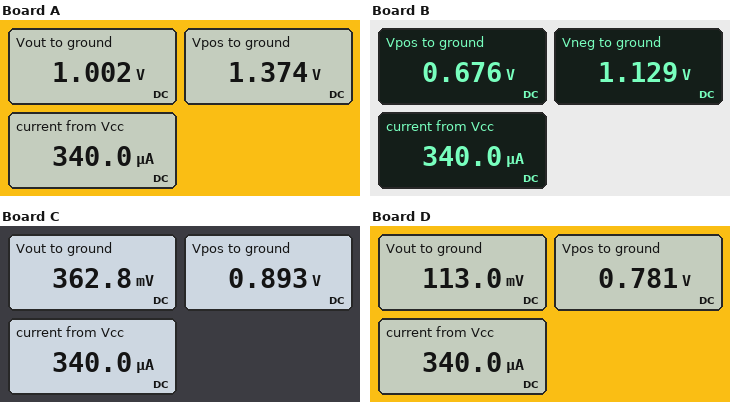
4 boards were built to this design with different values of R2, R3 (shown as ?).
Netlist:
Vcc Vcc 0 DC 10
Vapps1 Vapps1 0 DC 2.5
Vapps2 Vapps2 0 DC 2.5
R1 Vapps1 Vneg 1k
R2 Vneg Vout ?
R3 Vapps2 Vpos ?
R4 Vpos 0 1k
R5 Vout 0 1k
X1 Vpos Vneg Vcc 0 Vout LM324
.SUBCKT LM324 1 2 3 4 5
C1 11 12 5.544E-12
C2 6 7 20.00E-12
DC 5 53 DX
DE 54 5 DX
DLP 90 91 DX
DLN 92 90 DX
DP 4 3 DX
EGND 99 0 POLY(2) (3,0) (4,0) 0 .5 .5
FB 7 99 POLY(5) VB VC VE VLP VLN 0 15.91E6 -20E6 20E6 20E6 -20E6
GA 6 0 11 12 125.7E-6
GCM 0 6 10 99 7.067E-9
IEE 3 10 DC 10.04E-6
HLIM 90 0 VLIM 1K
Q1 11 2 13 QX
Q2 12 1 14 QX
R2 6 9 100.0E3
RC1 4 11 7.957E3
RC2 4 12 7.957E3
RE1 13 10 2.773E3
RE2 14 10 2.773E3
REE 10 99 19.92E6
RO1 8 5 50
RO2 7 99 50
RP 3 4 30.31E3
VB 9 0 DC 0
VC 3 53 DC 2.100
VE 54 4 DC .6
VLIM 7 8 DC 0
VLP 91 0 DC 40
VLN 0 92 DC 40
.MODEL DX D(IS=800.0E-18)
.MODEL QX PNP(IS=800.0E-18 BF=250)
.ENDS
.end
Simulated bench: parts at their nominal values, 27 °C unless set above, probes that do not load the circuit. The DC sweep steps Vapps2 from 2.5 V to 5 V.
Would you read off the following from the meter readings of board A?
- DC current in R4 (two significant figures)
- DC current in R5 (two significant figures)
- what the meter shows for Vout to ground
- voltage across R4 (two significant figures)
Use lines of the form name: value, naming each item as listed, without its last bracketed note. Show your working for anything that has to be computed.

DC current in R4: (1.374 V) / 1 kΩ = 1.4 mA
DC current in R5: (1.002 V) / 1 kΩ = 1.0 mA
what the meter shows for Vout to ground: 1.002 V
voltage across R4: 1.374 V = 1.4 V
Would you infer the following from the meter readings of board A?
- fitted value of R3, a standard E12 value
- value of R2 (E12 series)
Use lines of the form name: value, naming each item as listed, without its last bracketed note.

fitted value of R3, a standard E12 value: 820 Ω
value of R2: 330 Ω
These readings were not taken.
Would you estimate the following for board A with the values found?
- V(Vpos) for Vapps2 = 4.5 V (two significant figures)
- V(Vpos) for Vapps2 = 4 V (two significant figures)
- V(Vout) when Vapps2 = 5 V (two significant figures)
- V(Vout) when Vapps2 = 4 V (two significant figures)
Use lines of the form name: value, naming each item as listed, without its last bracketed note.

V(Vpos) for Vapps2 = 4.5 V: 2.5 V
V(Vpos) for Vapps2 = 4 V: 2.2 V
V(Vout) when Vapps2 = 5 V: 2.8 V
V(Vout) when Vapps2 = 4 V: 2.1 V
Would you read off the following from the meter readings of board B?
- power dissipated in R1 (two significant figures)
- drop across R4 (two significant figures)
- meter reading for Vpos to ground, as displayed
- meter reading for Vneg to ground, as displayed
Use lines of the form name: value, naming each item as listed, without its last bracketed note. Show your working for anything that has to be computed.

power dissipated in R1: (2.5 V - 1.129 V)^2 / 1 kΩ = 1.9 mW
drop across R4: 676 mV = 680 mV
meter reading for Vpos to ground, as displayed: 0.676 V
meter reading for Vneg to ground, as displayed: 1.129 V
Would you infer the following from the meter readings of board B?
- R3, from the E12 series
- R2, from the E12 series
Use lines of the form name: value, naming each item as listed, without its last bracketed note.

R3, from the E12 series: 2.7 kΩ
R2, from the E12 series: 820 Ω
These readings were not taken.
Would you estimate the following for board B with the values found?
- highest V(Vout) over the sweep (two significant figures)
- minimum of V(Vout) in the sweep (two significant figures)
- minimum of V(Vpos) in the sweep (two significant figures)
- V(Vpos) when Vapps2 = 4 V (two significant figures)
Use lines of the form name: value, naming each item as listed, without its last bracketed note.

highest V(Vout) over the sweep: 410 mV
minimum of V(Vout) in the sweep: 4.2 mV
minimum of V(Vpos) in the sweep: 680 mV
V(Vpos) when Vapps2 = 4 V: 1.1 V
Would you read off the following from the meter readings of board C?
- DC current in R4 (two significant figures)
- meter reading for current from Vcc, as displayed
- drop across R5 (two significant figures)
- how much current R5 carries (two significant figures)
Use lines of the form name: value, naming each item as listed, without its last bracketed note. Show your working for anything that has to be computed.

DC current in R4: (893 mV) / 1 kΩ = 890 µA
meter reading for current from Vcc, as displayed: 340.0 µA
drop across R5: 362.8 mV = 360 mV
how much current R5 carries: (362.8 mV) / 1 kΩ = 360 µA
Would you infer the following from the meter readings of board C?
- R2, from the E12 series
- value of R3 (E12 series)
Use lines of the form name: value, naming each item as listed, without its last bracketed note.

R2, from the E12 series: 330 Ω
value of R3: 1.8 kΩ
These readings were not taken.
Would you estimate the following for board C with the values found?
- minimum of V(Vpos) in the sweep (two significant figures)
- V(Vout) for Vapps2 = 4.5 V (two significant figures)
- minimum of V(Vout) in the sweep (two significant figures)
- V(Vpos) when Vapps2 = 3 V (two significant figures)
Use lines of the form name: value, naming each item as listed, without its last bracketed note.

minimum of V(Vpos) in the sweep: 890 mV
V(Vout) for Vapps2 = 4.5 V: 1.3 V
minimum of V(Vout) in the sweep: 360 mV
V(Vpos) when Vapps2 = 3 V: 1.1 V
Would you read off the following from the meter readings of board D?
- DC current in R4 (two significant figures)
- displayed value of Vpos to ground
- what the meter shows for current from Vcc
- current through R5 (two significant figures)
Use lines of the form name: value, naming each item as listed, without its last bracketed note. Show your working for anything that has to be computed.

DC current in R4: (781 mV) / 1 kΩ = 780 µA
displayed value of Vpos to ground: 0.781 V
what the meter shows for current from Vcc: 340.0 µA
current through R5: (113 mV) / 1 kΩ = 110 µA
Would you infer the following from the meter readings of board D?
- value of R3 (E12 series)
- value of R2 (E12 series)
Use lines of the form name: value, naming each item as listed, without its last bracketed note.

value of R3: 2.2 kΩ
value of R2: 390 Ω
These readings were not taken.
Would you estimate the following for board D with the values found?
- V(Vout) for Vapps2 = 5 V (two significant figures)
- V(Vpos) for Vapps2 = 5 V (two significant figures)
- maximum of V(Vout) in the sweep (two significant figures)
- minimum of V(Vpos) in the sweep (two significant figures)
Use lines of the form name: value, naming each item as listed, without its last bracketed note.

V(Vout) for Vapps2 = 5 V: 1.2 V
V(Vpos) for Vapps2 = 5 V: 1.6 V
maximum of V(Vout) in the sweep: 1.2 V
minimum of V(Vpos) in the sweep: 780 mV
